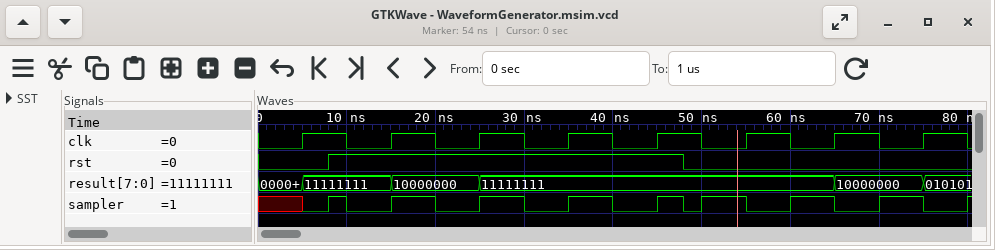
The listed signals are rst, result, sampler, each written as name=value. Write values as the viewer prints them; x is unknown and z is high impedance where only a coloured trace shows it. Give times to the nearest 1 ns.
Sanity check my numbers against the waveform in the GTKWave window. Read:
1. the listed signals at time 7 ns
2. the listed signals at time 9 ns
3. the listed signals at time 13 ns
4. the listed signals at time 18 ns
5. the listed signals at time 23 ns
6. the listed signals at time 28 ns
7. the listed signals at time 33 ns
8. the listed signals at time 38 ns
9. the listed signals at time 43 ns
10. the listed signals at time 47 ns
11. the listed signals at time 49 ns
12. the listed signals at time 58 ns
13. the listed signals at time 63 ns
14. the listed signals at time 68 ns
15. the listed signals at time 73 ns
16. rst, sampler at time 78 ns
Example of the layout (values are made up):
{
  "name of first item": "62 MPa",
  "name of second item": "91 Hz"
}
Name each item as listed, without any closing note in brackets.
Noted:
{
  "the listed signals at time 7 ns": "rst=0, result=11111111, sampler=0",
  "the listed signals at time 9 ns": "rst=1, result=11111111, sampler=1",
  "the listed signals at time 13 ns": "rst=1, result=11111111, sampler=0",
  "the listed signals at time 18 ns": "rst=1, result=10000000, sampler=1",
  "the listed signals at time 23 ns": "rst=1, result=10000000, sampler=0",
  "the listed signals at time 28 ns": "rst=1, result=11111111, sampler=1",
  "the listed signals at time 33 ns": "rst=1, result=11111111, sampler=0",
  "the listed signals at time 38 ns": "rst=1, result=11111111, sampler=1",
  "the listed signals at time 43 ns": "rst=1, result=11111111, sampler=0",
  "the listed signals at time 47 ns": "rst=1, result=11111111, sampler=1",
  "the listed signals at time 49 ns": "rst=0, result=11111111, sampler=0",
  "the listed signals at time 58 ns": "rst=0, result=11111111, sampler=0",
  "the listed signals at time 63 ns": "rst=0, result=11111111, sampler=1",
  "the listed signals at time 68 ns": "rst=0, result=10000000, sampler=0",
  "the listed signals at time 73 ns": "rst=0, result=10000000, sampler=1",
  "rst, sampler at time 78 ns": "rst=0, sampler=0"
}
